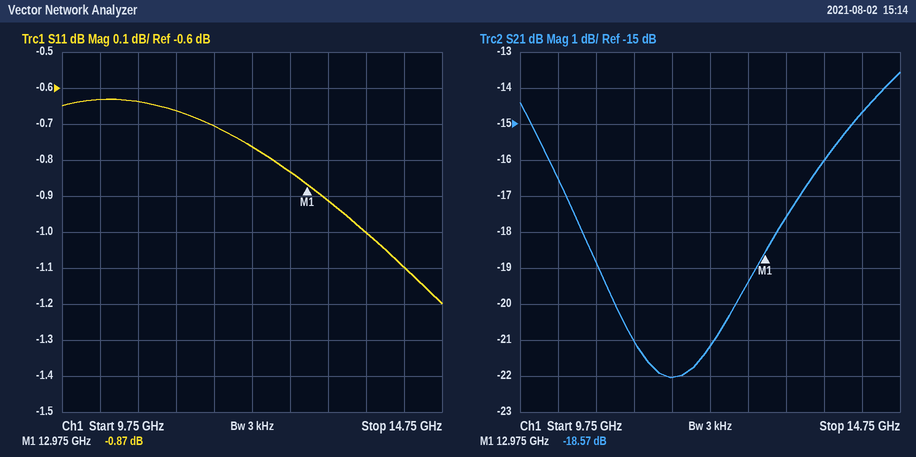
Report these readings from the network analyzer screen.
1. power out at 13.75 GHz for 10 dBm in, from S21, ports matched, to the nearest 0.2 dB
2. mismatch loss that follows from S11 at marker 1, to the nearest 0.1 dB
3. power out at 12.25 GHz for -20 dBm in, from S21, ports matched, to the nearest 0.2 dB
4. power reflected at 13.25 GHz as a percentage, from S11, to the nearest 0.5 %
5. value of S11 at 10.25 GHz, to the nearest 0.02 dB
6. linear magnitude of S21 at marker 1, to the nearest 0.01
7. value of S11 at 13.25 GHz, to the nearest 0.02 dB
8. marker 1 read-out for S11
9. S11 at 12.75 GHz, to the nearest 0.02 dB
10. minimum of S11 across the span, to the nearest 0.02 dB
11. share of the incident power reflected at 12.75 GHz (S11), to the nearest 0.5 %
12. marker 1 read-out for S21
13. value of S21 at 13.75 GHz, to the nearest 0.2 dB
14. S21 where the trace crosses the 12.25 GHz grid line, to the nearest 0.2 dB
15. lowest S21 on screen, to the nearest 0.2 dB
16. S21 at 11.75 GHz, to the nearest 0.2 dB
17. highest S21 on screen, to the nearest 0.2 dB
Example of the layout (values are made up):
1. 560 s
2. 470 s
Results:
1. -6.0 dBm
2. 7.4 dB
3. -41.2 dBm
4. 81.0 %
5. -0.64 dB
6. 0.12
7. -0.92 dB
8. -0.87 dB
9. -0.84 dB
10. -1.20 dB
11. 82.5 %
12. -18.57 dB
13. -16.0 dB
14. -21.2 dB
15. -22.0 dB
16. -22.0 dB
17. -13.6 dB
